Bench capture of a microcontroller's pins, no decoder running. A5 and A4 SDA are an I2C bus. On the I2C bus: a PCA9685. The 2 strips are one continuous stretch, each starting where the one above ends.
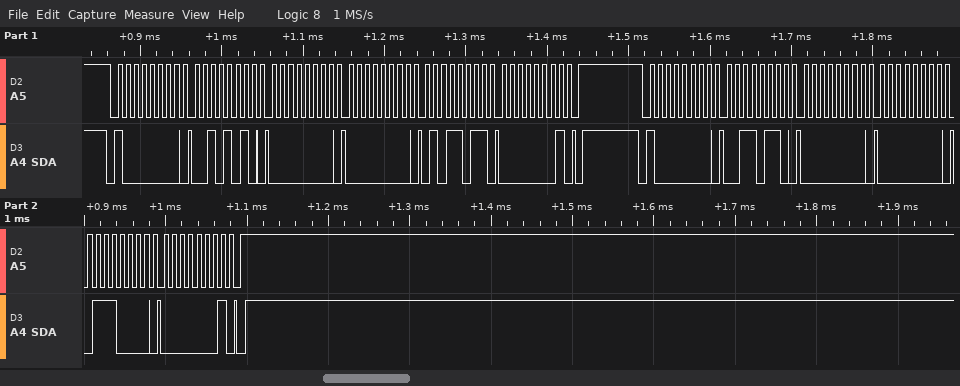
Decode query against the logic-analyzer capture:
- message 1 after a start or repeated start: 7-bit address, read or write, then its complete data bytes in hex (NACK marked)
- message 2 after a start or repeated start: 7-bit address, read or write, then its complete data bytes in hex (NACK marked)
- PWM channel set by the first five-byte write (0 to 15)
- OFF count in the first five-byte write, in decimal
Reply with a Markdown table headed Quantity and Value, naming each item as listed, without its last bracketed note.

| Quantity | Value |
|---|---|
| message 1 after a start or repeated start: 7-bit address, read or write, then its complete data bytes in hex | 0x40 write: 2A 00 00 5B 01 |
| message 2 after a start or repeated start: 7-bit address, read or write, then its complete data bytes in hex | 0x40 write: 36 00 00 70 01 |
| PWM channel set by the first five-byte write | 9 |
| OFF count in the first five-byte write, in decimal | 347 |
